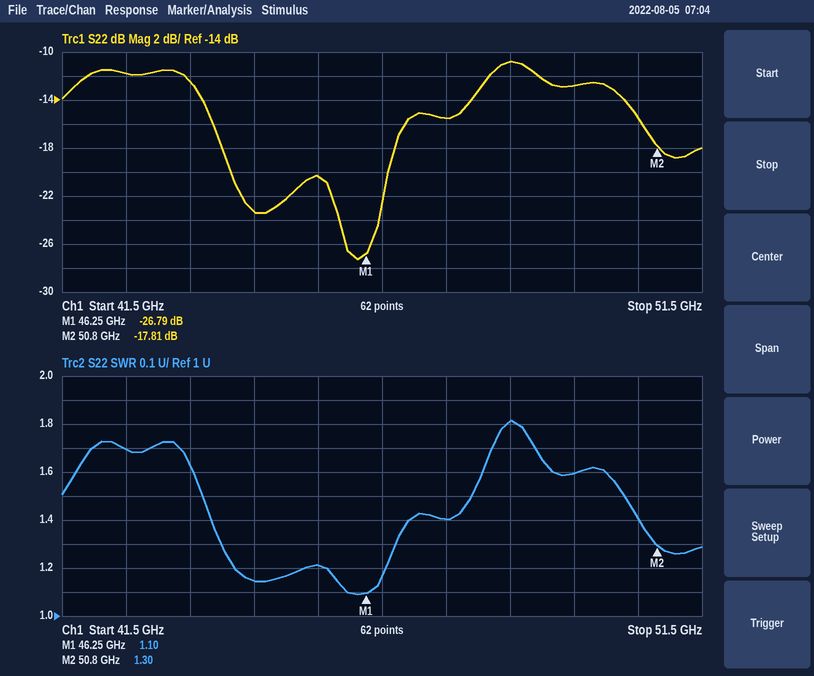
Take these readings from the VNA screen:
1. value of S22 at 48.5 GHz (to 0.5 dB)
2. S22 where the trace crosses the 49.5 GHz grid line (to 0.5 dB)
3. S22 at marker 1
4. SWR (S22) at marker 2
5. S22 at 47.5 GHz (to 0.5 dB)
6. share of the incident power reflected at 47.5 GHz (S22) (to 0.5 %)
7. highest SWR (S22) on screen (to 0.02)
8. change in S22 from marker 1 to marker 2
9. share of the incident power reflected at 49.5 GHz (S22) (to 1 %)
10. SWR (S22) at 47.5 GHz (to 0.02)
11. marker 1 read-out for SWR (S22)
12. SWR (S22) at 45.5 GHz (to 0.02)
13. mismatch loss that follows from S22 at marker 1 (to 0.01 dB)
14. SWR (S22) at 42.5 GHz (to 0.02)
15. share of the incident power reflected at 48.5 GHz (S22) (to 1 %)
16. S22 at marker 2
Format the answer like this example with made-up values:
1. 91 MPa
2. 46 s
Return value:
1. -11.0 dB
2. -13.0 dB
3. -26.79 dB
4. 1.30
5. -15.5 dB
6. 3.0 %
7. 1.82
8. 8.98 dB
9. 5 %
10. 1.40
11. 1.10
12. 1.22
13. 0.01 dB
14. 1.70
15. 8 %
16. -17.81 dB
